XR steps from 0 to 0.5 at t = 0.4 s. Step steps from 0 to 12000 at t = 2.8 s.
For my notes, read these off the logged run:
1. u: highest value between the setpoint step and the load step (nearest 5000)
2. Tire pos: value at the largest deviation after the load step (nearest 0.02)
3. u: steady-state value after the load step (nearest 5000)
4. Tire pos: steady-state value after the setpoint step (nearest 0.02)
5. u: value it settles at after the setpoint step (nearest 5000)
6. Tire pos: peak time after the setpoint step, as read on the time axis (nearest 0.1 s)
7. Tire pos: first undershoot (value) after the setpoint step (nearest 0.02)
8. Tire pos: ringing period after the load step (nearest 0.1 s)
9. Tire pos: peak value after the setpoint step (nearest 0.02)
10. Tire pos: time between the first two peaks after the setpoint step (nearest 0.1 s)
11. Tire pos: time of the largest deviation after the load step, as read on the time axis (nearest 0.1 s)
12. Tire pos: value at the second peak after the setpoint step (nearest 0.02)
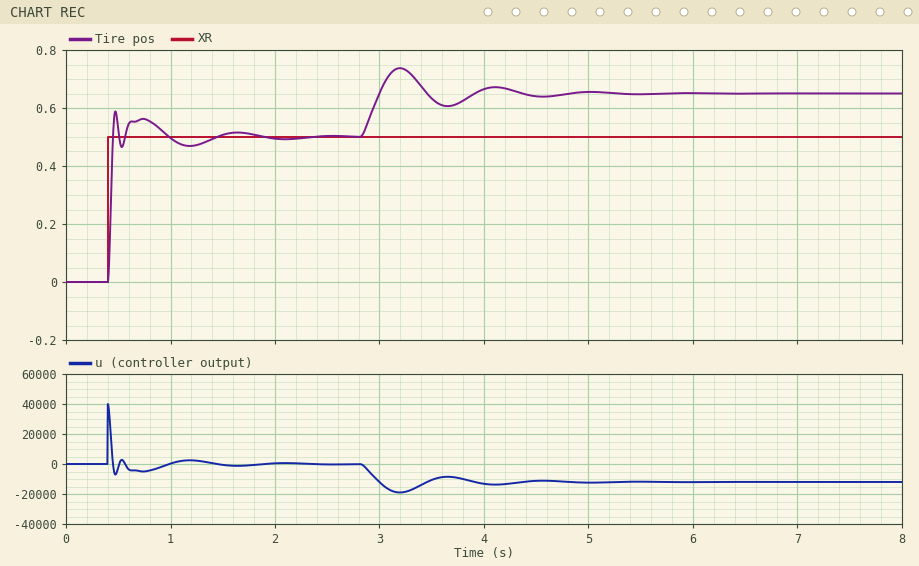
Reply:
40000
0.74
-10000
0.50
0
0.5 s
0.46
0.9 s
0.58
0.3 s
3.2 s
0.56
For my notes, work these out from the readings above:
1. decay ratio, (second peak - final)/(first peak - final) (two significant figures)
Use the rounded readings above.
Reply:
0.75
